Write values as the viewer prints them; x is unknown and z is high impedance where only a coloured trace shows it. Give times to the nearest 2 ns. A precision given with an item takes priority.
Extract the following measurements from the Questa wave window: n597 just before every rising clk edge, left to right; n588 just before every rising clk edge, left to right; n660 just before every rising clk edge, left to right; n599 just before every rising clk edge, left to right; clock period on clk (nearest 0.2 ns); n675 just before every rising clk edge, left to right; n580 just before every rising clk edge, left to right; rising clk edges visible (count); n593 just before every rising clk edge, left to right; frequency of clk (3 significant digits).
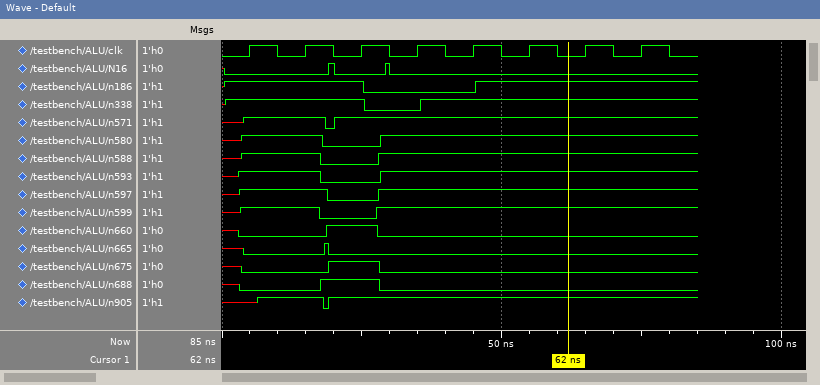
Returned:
1 1 0 1 1 1 1 1
1 1 0 1 1 1 1 1
0 0 1 0 0 0 0 0
1 1 0 1 1 1 1 1
10 ns
0 0 1 0 0 0 0 0
1 1 0 1 1 1 1 1
8
1 1 0 1 1 1 1 1
100 MHz
